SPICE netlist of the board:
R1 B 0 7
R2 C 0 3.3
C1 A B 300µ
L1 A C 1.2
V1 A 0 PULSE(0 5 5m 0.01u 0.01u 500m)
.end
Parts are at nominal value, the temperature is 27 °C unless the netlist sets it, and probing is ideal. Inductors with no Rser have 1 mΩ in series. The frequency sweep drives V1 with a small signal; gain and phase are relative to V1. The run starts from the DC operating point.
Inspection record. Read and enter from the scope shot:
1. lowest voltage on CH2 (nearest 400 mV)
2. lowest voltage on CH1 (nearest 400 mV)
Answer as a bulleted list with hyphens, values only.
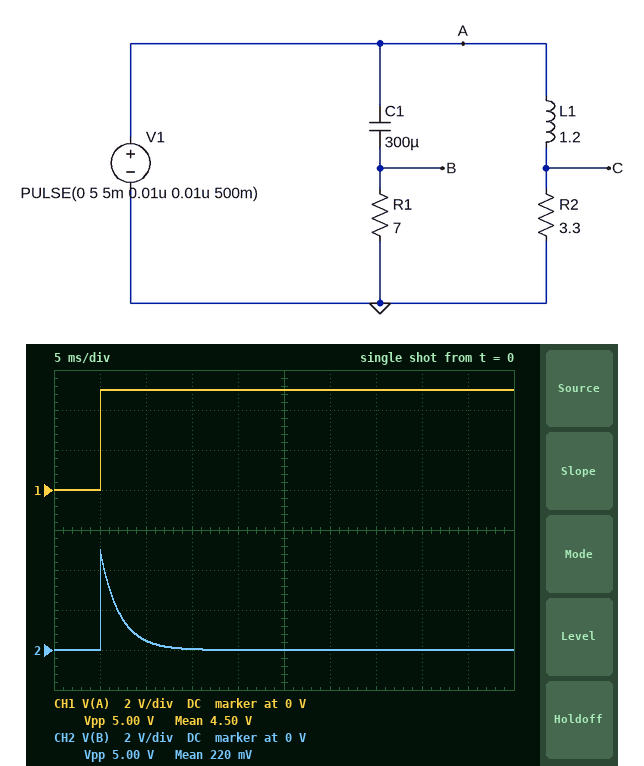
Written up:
- 0 V
- 0 V
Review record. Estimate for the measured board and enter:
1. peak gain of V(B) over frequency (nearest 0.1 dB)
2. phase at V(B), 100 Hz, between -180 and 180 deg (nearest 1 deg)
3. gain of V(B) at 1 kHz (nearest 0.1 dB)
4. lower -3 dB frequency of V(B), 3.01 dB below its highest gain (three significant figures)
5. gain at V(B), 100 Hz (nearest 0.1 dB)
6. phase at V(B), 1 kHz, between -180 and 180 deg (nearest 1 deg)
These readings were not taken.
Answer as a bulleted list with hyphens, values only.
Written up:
- 0 dB
- 37 deg
- 0 dB
- 75.8 Hz
- -2.0 dB
- 4 deg
